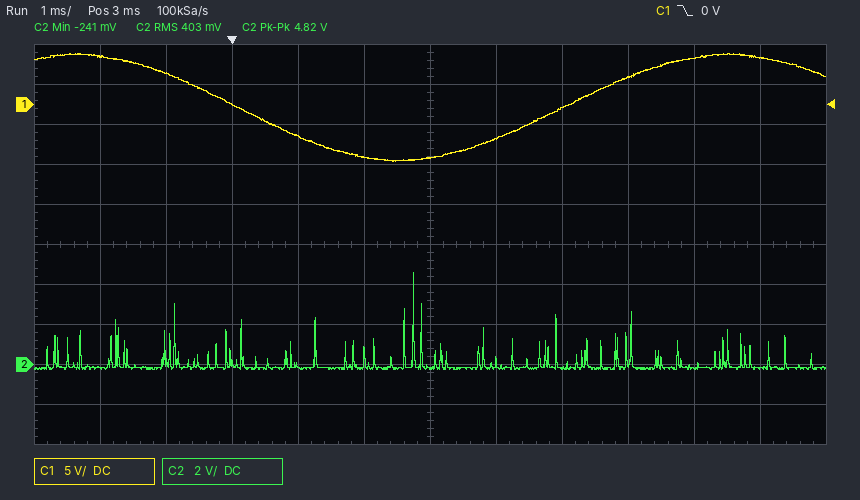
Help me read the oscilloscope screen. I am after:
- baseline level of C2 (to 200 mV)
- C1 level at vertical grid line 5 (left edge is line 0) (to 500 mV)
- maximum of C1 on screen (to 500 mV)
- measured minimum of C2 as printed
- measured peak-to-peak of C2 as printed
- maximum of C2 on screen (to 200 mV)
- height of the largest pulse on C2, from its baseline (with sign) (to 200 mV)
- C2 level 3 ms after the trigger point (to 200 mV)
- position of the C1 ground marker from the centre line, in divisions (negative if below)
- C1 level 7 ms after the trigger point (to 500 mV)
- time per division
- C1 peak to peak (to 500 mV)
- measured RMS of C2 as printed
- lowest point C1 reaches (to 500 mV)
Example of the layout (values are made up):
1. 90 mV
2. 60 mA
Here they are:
1. -200 mV
2. -6.5 V
3. 6.5 V
4. -241 mV
5. 4.82 V
6. 4.6 V
7. +4.8 V
8. -200 mV
9. +3.5 div
10. 6.0 V
11. 1 ms
12. 13.5 V
13. 403 mV
14. -7.0 V
